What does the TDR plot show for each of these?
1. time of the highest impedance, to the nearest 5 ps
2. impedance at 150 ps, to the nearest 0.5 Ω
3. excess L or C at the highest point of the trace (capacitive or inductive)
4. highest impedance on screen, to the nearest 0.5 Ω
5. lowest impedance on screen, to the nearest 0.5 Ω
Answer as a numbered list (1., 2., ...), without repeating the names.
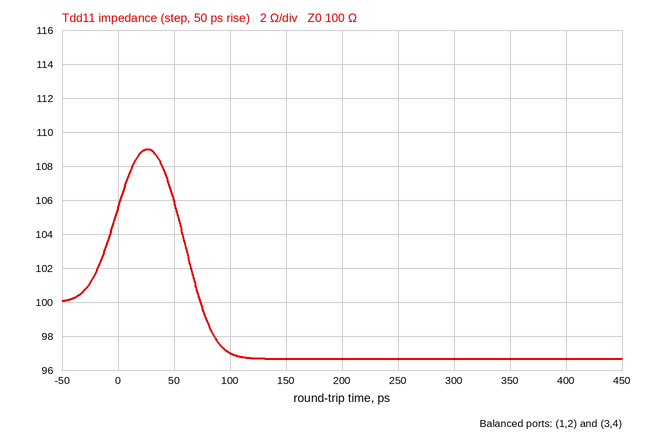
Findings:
1. 25 ps
2. 96.5 Ω
3. inductive
4. 109.0 Ω
5. 96.5 Ω
